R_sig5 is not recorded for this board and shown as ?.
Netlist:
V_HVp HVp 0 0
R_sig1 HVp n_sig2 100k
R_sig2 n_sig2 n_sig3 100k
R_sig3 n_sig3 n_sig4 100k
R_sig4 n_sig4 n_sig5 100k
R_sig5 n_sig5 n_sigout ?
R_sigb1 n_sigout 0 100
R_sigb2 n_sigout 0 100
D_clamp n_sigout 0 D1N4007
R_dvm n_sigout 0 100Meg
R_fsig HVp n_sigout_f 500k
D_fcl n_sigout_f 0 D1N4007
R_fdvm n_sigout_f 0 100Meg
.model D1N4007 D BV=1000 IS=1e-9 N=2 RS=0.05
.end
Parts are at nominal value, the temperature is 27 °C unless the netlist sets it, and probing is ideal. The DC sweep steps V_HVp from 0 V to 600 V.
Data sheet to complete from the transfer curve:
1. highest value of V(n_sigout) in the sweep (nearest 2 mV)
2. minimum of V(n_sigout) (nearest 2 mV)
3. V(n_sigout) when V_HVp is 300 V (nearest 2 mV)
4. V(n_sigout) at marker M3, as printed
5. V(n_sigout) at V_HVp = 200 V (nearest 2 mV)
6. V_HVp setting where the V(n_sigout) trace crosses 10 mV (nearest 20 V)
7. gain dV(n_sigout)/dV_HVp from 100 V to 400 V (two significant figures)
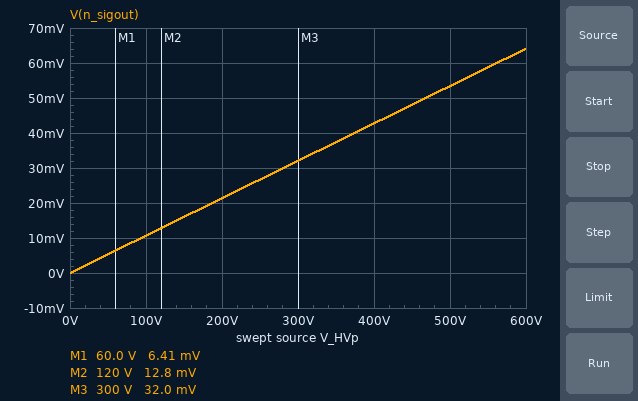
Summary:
64 mV
0 V
32 mV
32.0 mV
22 mV
100 V
0.00011 V/V
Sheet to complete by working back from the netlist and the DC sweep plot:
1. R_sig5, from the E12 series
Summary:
68 kΩ
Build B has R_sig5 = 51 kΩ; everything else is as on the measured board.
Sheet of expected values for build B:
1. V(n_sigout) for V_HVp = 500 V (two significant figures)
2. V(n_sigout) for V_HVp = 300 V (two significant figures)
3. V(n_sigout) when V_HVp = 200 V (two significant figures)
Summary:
55 mV
33 mV
22 mV
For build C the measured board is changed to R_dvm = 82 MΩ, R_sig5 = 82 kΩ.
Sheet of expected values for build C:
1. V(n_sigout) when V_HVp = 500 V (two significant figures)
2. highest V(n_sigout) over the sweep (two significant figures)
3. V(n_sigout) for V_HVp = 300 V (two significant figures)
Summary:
52 mV
62 mV
31 mV
